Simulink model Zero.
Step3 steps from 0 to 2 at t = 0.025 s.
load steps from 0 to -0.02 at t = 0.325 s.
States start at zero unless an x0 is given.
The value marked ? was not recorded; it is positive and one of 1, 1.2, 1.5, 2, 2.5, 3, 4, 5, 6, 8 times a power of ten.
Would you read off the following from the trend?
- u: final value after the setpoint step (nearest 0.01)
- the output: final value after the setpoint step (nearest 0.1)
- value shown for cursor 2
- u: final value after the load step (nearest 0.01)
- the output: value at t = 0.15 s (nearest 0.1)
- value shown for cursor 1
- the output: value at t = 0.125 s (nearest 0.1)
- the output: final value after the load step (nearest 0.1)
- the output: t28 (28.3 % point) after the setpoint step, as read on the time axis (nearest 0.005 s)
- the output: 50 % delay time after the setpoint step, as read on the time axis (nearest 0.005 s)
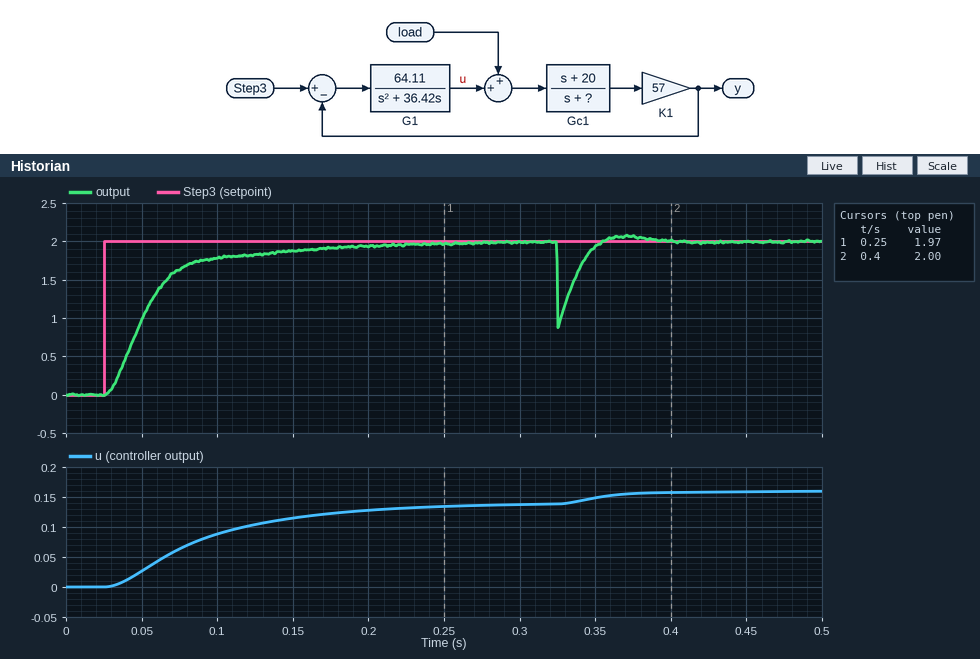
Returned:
0.14
2.0
2.00
0.16
1.9
1.97
1.8
2.0
0.040 s
0.050 s
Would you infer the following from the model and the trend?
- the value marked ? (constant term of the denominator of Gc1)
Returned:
80
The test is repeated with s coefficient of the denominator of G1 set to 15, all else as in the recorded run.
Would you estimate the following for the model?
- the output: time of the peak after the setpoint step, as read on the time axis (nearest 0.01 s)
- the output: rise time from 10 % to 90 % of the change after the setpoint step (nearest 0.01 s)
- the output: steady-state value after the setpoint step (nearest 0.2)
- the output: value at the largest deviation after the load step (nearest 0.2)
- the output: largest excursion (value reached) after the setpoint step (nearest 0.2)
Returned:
0.09 s
0.03 s
2.0
0.8
2.2
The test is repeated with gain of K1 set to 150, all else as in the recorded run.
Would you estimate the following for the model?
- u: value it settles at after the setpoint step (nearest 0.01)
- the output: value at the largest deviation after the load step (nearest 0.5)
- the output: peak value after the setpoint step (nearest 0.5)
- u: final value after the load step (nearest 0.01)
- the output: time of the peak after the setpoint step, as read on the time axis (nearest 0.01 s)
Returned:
0.05
-1.0
2.0
0.07
0.06 s
